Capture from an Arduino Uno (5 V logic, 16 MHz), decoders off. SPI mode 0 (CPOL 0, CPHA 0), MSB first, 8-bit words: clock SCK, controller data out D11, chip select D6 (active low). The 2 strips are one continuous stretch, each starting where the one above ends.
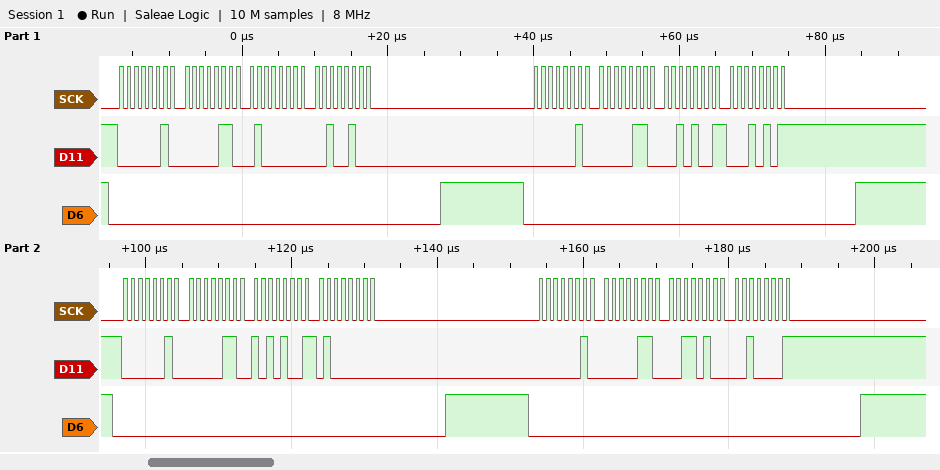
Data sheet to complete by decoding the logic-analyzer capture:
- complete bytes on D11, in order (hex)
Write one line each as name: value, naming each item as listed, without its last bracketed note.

complete bytes on D11, in order: 02 06 40 24 02 06 29 15 02 06 A9 40 02 06 34 21
